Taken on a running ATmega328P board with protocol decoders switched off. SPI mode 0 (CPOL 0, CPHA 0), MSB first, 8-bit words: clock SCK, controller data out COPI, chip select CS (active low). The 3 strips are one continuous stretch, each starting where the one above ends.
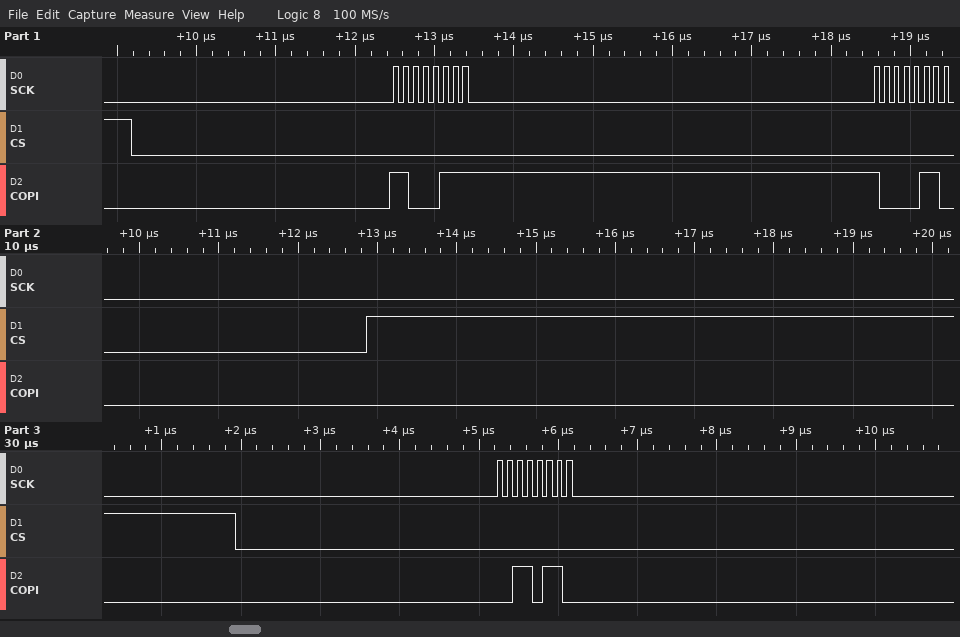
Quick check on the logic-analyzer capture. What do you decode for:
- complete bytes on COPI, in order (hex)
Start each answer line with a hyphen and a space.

- C7 86 36
